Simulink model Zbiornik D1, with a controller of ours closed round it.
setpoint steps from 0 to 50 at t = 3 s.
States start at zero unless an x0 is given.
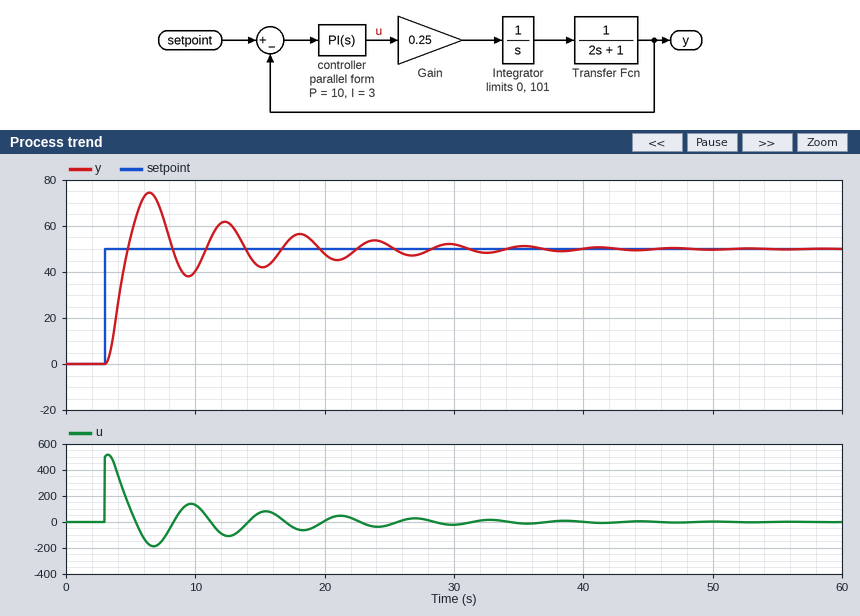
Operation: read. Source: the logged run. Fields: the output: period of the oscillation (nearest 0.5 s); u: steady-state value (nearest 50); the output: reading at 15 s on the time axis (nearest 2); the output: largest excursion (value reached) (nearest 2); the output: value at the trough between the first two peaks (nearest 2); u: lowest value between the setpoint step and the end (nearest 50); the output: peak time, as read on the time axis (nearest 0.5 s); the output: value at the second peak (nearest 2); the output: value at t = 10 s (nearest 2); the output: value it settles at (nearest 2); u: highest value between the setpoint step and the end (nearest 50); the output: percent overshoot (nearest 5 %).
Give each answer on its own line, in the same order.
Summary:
6.0 s
0
42
74
38
-200
6.5 s
62
40
50
500
50 %
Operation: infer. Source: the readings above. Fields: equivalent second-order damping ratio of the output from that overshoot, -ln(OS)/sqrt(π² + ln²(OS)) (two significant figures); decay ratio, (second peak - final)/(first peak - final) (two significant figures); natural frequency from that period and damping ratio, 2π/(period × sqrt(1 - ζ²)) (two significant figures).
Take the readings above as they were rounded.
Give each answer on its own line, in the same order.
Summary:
0.22
0.50
1.1 rad/s
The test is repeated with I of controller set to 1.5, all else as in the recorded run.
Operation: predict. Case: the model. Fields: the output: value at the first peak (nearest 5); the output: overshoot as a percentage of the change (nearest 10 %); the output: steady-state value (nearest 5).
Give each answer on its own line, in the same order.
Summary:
70
40 %
50
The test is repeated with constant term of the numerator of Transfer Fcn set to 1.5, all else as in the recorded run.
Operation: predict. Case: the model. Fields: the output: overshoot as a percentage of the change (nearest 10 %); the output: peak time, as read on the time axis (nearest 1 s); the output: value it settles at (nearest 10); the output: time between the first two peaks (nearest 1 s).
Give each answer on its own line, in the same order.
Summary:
70 %
5 s
50
5 s
